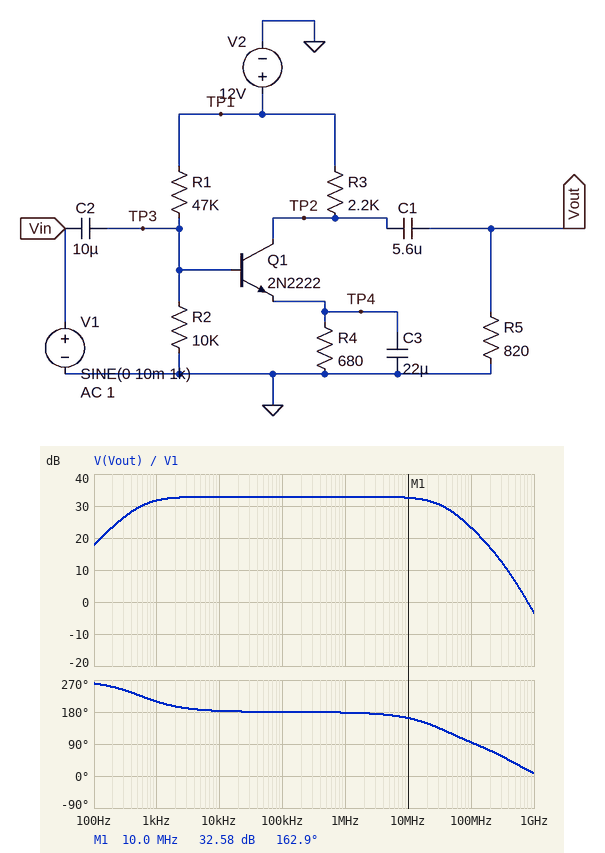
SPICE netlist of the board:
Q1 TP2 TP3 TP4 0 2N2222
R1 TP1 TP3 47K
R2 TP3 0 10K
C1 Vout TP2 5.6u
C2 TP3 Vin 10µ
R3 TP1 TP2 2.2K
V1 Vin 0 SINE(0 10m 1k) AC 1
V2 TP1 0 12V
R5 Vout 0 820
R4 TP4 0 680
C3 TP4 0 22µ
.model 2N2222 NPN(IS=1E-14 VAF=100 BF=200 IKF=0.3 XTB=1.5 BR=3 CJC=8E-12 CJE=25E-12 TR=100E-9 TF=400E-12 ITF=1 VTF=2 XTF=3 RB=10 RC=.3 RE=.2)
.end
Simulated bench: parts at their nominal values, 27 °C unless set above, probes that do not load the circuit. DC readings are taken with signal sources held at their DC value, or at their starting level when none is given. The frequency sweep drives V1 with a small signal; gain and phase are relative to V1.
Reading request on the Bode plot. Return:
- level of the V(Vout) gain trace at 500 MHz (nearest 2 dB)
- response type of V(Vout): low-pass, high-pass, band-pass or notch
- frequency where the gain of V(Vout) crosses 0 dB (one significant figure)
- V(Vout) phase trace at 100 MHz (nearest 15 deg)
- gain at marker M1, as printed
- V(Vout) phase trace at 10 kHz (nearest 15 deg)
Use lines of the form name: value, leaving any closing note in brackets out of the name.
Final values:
level of the V(Vout) gain trace at 500 MHz: 6 dB
response type of V(Vout): low-pass, high-pass, band-pass or notch: band-pass
frequency where the gain of V(Vout) crosses 0 dB: 800 MHz
V(Vout) phase trace at 100 MHz: 90 deg
gain at marker M1, as printed: 32.58 dB
V(Vout) phase trace at 10 kHz: 180 deg
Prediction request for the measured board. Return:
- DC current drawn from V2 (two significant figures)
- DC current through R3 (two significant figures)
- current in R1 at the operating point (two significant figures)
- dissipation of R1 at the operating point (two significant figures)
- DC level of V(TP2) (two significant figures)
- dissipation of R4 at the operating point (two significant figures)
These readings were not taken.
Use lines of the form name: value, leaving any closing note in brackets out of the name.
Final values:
DC current drawn from V2: 2.2 mA
DC current through R3: 2.0 mA
current in R1 at the operating point: 210 µA
dissipation of R1 at the operating point: 2.1 mW
DC level of V(TP2): 7.6 V
dissipation of R4 at the operating point: 2.7 mW
